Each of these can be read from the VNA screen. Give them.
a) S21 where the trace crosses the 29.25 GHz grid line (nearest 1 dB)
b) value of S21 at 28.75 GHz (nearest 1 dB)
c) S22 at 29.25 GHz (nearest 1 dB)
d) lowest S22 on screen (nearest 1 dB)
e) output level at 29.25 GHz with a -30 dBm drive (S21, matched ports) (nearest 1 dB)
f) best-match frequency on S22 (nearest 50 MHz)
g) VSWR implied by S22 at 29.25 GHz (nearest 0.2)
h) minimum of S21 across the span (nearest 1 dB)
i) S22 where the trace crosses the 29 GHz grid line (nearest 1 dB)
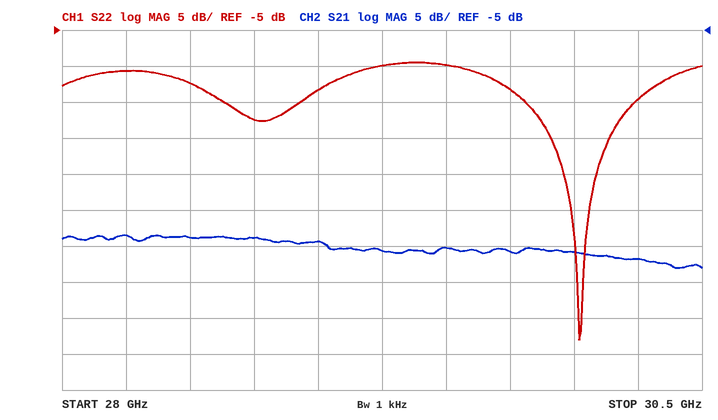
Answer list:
-36 dB
-34 dB
-10 dB
-48 dB
-66 dBm
30.00 GHz
2.0
-38 dB
-13 dB
